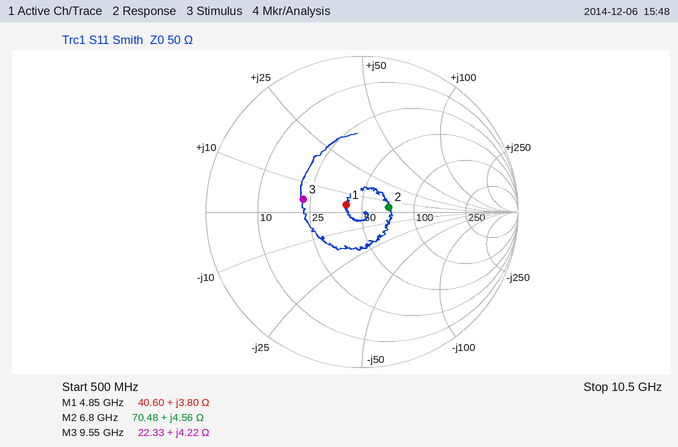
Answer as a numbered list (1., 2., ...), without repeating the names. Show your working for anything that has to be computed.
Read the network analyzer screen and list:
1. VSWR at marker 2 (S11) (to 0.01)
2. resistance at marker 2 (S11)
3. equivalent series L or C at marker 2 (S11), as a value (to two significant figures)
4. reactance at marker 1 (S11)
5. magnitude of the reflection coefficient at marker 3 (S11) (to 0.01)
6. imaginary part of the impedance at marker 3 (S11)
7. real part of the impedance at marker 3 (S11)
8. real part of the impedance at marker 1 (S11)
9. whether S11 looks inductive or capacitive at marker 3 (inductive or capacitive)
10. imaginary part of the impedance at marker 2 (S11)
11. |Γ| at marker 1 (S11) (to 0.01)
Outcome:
1. 1.42
2. 70.48 Ω
3. L = 4.56 Ω/(2π × 6.8 GHz) ≈ 107 pH, so 110 pH to two significant figures
4. +3.80 Ω
5. 0.39
6. +4.22 Ω
7. 22.33 Ω
8. 40.60 Ω
9. inductive
10. +4.56 Ω
11. 0.11
